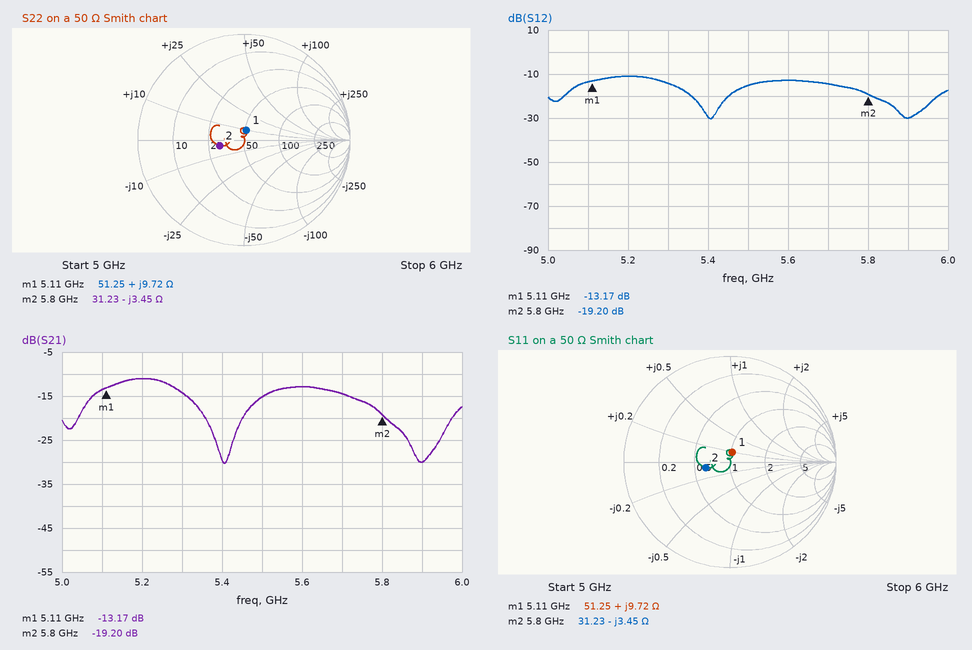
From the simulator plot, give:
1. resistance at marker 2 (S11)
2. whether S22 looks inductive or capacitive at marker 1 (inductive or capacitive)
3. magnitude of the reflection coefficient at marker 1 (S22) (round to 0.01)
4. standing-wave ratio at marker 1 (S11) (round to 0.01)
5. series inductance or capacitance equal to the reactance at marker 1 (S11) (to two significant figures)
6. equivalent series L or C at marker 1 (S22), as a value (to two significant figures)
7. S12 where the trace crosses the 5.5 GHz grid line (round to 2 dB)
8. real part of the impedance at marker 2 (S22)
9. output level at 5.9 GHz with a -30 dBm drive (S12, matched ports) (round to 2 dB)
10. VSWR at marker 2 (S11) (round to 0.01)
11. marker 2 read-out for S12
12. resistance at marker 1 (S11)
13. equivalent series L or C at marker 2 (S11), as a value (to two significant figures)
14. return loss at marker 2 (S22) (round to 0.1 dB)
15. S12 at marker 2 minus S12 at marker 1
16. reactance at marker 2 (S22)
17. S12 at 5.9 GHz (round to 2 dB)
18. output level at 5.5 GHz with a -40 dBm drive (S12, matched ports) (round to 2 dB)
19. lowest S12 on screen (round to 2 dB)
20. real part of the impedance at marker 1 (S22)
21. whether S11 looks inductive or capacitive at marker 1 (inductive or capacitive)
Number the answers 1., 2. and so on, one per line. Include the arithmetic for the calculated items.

1. 31.23 Ω
2. inductive
3. 0.10
4. 1.21
5. L = 9.72 Ω/(2π × 5.11 GHz) ≈ 303 pH, so 300 pH to two significant figures
6. L = 9.72 Ω/(2π × 5.11 GHz) ≈ 303 pH, so 300 pH to two significant figures
7. -16 dB
8. 31.23 Ω
9. -30 dBm + (-30 dB) = -60 dBm
10. 1.61
11. -19.20 dB
12. 51.25 Ω
13. C = 1/(2π × 5.8 GHz × 3.45 Ω) ≈ 8.0 pF
14. 12.6 dB
15. -19.2 − (-13.17) = -6.03 dB
16. -3.45 Ω
17. -30 dB
18. -40 dBm + (-16 dB) = -56 dBm
19. -30 dB
20. 51.25 Ω
21. inductive
